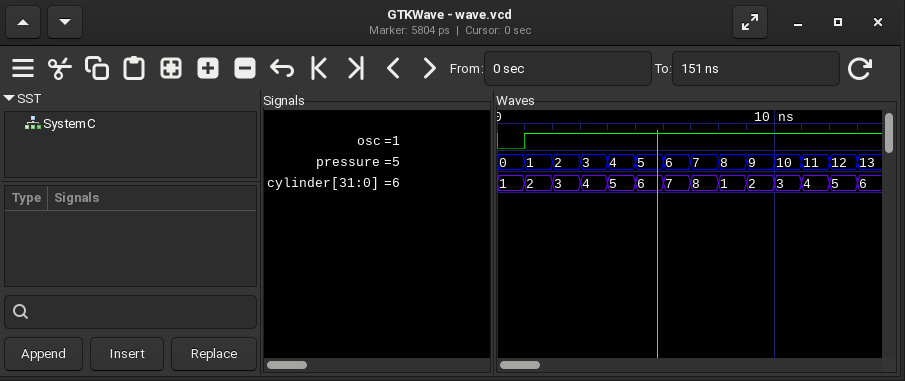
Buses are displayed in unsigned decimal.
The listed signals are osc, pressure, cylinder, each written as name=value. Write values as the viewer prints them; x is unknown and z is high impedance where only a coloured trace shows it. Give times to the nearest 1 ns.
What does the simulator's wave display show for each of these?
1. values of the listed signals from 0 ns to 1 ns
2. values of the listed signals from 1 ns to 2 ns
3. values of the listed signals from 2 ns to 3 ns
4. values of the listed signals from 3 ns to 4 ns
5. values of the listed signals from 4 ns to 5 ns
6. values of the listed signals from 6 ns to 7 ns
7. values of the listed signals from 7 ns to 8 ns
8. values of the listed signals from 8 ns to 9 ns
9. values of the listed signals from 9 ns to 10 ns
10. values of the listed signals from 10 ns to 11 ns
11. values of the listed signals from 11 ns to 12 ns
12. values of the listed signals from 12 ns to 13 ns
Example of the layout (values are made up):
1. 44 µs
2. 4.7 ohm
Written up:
1. osc=0, pressure=0, cylinder=1
2. osc=1, pressure=1, cylinder=2
3. osc=1, pressure=2, cylinder=3
4. osc=1, pressure=3, cylinder=4
5. osc=1, pressure=4, cylinder=5
6. osc=1, pressure=6, cylinder=7
7. osc=1, pressure=7, cylinder=8
8. osc=1, pressure=8, cylinder=1
9. osc=1, pressure=9, cylinder=2
10. osc=1, pressure=10, cylinder=3
11. osc=1, pressure=11, cylinder=4
12. osc=1, pressure=12, cylinder=5
